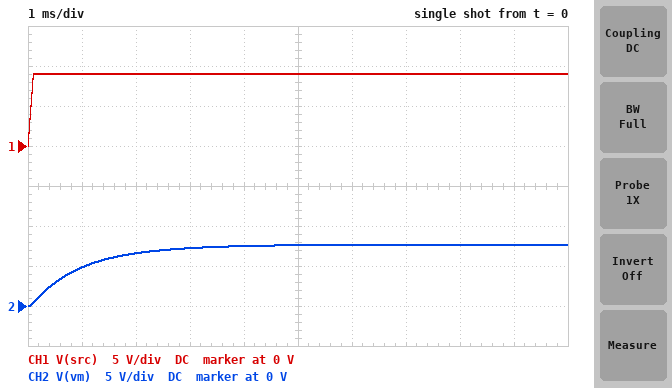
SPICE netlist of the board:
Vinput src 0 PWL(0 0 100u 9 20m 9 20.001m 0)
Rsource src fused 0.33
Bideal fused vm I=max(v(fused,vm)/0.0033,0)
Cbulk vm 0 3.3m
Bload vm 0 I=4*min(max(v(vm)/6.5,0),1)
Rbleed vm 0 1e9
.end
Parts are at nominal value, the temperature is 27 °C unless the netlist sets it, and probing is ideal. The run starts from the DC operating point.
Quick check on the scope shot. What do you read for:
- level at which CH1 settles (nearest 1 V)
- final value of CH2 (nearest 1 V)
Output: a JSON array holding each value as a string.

["9 V", "8 V"]
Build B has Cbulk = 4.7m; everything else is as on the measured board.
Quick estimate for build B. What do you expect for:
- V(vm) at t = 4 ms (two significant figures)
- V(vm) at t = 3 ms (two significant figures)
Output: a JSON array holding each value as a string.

["7.2 V", "6.7 V"]
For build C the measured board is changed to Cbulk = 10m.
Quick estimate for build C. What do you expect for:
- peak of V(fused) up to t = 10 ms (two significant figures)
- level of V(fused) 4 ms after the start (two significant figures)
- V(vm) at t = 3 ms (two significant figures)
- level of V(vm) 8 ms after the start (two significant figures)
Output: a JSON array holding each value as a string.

["7.4 V", "5.7 V", "4.9 V", "7.1 V"]
